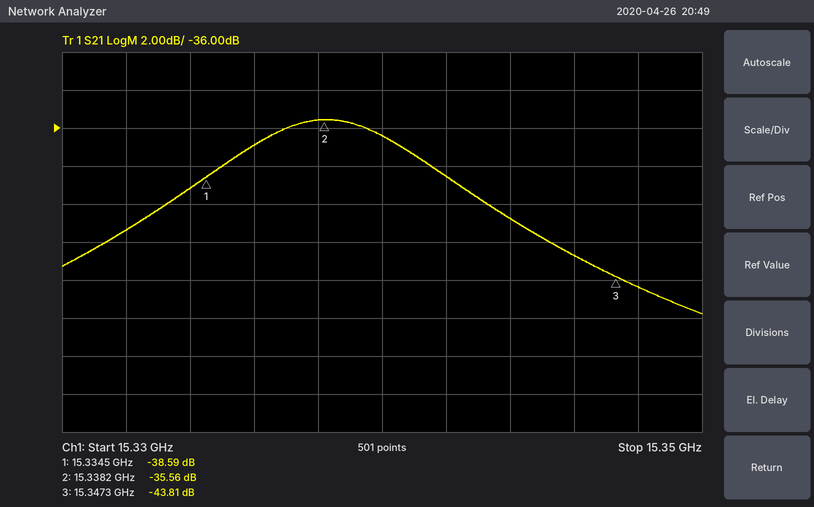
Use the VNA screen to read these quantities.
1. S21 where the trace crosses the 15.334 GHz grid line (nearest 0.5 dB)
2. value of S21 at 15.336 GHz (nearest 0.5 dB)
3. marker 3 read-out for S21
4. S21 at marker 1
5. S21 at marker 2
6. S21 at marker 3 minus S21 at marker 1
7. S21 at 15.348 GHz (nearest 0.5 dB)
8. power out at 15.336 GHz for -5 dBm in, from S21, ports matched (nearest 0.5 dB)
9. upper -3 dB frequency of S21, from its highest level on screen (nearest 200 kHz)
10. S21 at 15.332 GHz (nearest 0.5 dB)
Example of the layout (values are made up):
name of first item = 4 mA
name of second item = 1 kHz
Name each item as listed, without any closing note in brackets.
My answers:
S21 where the trace crosses the 15.334 GHz grid line = -39.0 dB
value of S21 at 15.336 GHz = -37.0 dB
marker 3 read-out for S21 = -43.81 dB
S21 at marker 1 = -38.59 dB
S21 at marker 2 = -35.56 dB
S21 at marker 3 minus S21 at marker 1 = -5.22 dB
S21 at 15.348 GHz = -44.5 dB
power out at 15.336 GHz for -5 dBm in, from S21, ports matched = -42.0 dBm
upper -3 dB frequency of S21, from its highest level on screen = 15.3420 GHz
S21 at 15.332 GHz = -41.5 dB
